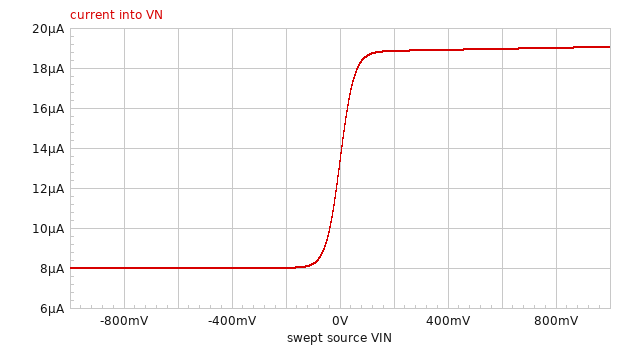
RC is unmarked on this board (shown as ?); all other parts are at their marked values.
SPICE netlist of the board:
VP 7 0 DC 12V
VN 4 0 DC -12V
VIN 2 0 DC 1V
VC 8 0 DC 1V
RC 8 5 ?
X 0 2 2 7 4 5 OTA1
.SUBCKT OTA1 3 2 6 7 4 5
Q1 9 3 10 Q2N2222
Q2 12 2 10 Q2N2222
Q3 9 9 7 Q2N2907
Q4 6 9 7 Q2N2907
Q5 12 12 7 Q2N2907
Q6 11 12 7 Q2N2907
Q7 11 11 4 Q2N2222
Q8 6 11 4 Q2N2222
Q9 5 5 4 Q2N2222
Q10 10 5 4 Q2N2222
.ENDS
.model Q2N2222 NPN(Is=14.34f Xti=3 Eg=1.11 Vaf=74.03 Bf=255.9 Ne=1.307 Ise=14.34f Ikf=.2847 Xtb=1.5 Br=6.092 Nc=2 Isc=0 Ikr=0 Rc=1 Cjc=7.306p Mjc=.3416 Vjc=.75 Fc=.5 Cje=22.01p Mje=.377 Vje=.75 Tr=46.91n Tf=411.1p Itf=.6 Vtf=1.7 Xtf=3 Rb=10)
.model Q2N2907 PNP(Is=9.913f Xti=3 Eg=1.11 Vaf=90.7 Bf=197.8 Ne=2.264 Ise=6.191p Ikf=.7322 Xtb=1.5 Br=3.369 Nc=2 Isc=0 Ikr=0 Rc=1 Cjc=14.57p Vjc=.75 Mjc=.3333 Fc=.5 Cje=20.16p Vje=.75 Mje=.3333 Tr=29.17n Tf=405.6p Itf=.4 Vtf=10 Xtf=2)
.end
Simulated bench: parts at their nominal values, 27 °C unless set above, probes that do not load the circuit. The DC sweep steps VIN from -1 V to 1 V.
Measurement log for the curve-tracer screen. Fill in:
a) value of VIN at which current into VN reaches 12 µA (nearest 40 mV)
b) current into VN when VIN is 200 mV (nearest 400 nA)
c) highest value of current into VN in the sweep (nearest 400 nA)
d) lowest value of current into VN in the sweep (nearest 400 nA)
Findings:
0 V
18.8 µA
19.2 µA
8.0 µA
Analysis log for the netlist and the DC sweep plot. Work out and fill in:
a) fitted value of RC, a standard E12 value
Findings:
3.3 MΩ
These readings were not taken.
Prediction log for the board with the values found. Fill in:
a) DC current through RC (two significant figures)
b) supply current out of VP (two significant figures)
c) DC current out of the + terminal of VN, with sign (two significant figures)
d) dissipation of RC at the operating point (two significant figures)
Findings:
3.8 µA
9.4 µA
-19 µA
47 µW
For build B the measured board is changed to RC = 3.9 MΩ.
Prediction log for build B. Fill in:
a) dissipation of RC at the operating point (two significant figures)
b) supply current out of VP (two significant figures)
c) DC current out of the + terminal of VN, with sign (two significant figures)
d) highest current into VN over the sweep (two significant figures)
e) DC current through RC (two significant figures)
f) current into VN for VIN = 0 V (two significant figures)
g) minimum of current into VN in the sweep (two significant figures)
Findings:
40 µW
7.9 µA
-16 µA
16 µA
3.2 µA
11 µA
6.8 µA
